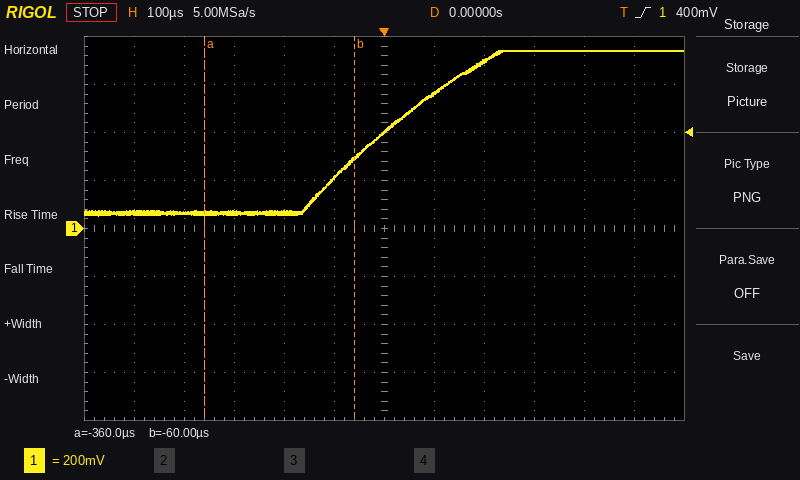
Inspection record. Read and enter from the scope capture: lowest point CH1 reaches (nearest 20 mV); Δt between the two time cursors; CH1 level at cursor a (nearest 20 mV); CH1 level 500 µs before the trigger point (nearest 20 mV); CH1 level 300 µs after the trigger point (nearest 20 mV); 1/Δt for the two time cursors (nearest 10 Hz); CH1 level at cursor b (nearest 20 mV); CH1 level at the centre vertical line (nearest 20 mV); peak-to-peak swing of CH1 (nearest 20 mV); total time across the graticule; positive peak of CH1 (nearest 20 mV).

60 mV
300 µs
60 mV
60 mV
740 mV
3.33 kHz
300 mV
400 mV
680 mV
1.2 ms
740 mV
